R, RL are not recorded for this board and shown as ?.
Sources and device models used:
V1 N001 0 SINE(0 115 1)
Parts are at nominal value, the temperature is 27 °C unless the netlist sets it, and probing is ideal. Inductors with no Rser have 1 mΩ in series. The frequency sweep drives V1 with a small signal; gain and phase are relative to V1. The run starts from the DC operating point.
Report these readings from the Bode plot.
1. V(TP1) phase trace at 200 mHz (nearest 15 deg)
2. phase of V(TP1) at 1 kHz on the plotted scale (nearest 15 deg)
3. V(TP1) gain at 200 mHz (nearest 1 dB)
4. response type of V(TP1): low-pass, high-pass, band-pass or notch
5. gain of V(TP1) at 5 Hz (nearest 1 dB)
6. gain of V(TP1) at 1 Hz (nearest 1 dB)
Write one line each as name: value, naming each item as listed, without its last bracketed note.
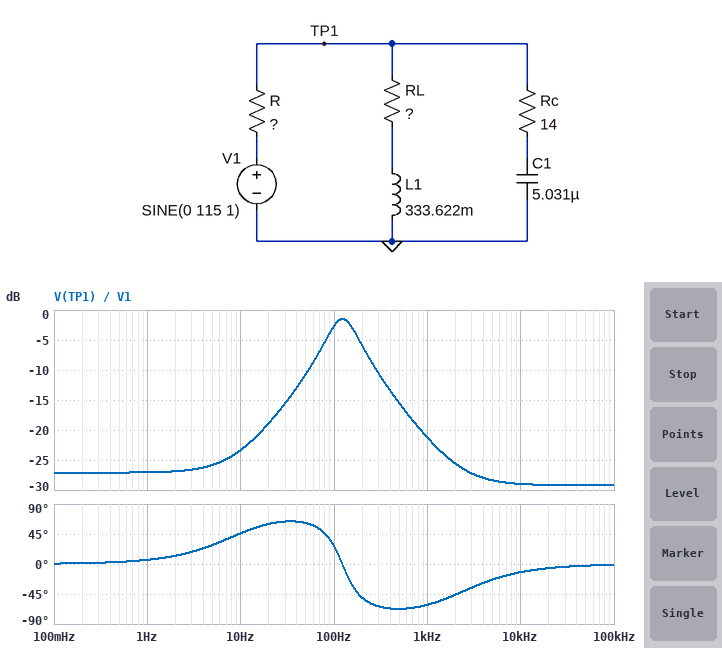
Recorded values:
V(TP1) phase trace at 200 mHz: 0 deg
phase of V(TP1) at 1 kHz on the plotted scale: -60 deg
V(TP1) gain at 200 mHz: -27 dB
response type of V(TP1): low-pass, high-pass, band-pass or notch: band-pass
gain of V(TP1) at 5 Hz: -26 dB
gain of V(TP1) at 1 Hz: -27 dB
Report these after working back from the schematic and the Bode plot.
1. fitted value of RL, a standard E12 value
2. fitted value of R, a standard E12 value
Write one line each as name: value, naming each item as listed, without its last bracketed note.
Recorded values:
fitted value of RL, a standard E12 value: 18 Ω
fitted value of R, a standard E12 value: 390 Ω
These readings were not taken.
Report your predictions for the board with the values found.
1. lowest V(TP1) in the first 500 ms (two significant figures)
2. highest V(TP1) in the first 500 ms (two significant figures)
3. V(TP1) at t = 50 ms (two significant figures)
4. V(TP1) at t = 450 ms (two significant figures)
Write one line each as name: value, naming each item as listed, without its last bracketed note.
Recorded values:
lowest V(TP1) in the first 500 ms: -560 mV
highest V(TP1) in the first 500 ms: 5.1 V
V(TP1) at t = 50 ms: 2.1 V
V(TP1) at t = 450 ms: 1.0 V
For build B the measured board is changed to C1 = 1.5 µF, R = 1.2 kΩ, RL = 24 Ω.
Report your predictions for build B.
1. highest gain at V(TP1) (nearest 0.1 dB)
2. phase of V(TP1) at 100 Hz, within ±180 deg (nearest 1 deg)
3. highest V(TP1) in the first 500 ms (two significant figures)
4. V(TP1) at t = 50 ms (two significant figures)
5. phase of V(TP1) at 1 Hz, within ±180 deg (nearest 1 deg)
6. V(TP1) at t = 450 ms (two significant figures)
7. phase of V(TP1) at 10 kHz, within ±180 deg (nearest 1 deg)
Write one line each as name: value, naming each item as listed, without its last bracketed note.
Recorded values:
highest gain at V(TP1): -1.6 dB
phase of V(TP1) at 100 Hz, within ±180 deg: 70 deg
highest V(TP1) in the first 500 ms: 2.3 V
V(TP1) at t = 50 ms: 880 mV
phase of V(TP1) at 1 Hz, within ±180 deg: 5 deg
V(TP1) at t = 450 ms: 510 mV
phase of V(TP1) at 10 kHz, within ±180 deg: -37 deg
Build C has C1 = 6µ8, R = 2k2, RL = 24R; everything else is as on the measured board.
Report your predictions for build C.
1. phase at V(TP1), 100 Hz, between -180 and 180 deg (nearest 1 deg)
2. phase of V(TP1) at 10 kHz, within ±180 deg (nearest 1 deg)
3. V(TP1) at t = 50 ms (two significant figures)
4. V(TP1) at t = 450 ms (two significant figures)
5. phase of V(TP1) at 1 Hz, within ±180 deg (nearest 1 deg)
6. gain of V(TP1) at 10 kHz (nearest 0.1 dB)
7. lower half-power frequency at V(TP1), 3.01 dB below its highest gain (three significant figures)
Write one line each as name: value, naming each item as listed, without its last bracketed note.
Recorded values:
phase at V(TP1), 100 Hz, between -180 and 180 deg: 20 deg
phase of V(TP1) at 10 kHz, within ±180 deg: -9 deg
V(TP1) at t = 50 ms: 480 mV
V(TP1) at t = 450 ms: 280 mV
phase of V(TP1) at 1 Hz, within ±180 deg: 5 deg
gain of V(TP1) at 10 kHz: -43.9 dB
lower half-power frequency at V(TP1), 3.01 dB below its highest gain: 92.5 Hz
